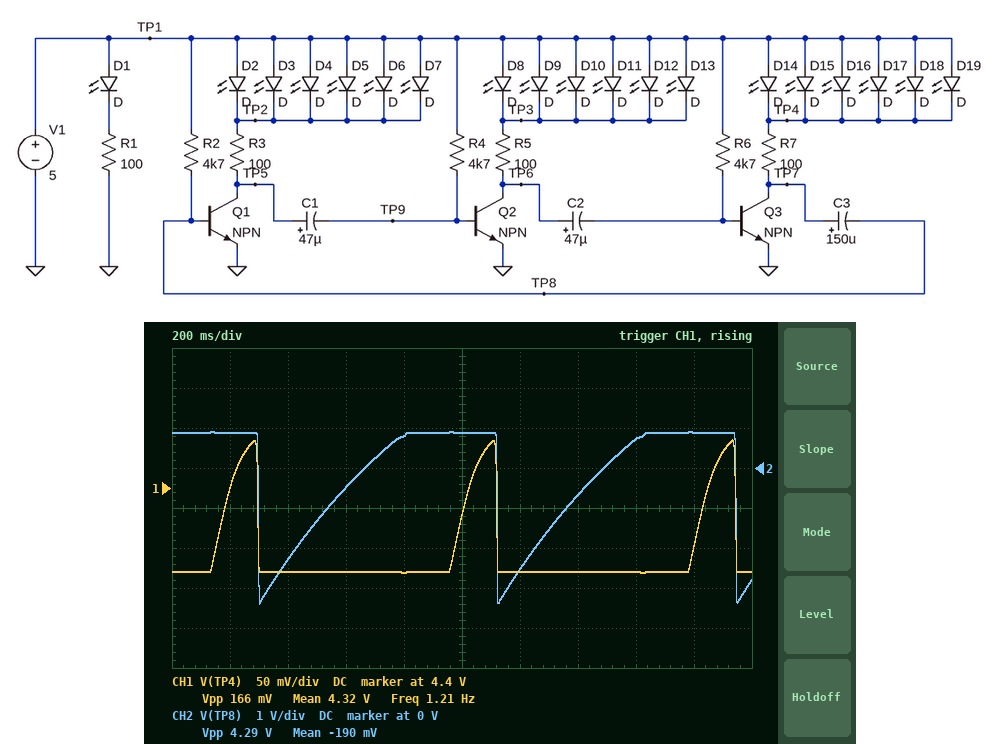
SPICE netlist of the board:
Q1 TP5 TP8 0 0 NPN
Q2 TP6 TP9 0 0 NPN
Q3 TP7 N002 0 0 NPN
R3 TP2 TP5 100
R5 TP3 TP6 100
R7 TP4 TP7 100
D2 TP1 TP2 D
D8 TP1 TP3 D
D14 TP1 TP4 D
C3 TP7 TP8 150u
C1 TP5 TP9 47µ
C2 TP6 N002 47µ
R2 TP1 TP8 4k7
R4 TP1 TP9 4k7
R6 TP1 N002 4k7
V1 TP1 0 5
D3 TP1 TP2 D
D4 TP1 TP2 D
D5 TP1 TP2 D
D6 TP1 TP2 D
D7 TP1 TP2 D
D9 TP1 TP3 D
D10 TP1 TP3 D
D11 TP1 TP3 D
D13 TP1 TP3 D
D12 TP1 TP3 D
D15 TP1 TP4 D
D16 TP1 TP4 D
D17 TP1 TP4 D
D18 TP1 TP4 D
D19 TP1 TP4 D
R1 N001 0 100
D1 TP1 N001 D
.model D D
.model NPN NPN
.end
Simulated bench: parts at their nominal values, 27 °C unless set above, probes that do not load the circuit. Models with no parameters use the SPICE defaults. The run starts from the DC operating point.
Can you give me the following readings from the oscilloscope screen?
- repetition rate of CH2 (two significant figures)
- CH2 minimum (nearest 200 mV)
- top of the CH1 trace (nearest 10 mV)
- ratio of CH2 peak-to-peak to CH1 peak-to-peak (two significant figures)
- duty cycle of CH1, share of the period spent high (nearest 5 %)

1.2 Hz
-3.4 V
4.46 V
26
15 %
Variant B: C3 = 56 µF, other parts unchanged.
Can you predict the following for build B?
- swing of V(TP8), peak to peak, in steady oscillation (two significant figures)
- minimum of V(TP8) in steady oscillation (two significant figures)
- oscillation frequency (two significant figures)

4.2 V
-3.3 V
2.0 Hz
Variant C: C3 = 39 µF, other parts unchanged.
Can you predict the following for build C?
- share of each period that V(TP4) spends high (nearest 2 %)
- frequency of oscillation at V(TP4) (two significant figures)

32 %
2.2 Hz
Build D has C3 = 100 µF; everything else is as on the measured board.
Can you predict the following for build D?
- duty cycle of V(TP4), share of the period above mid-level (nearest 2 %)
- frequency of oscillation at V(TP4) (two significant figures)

18 %
1.5 Hz
